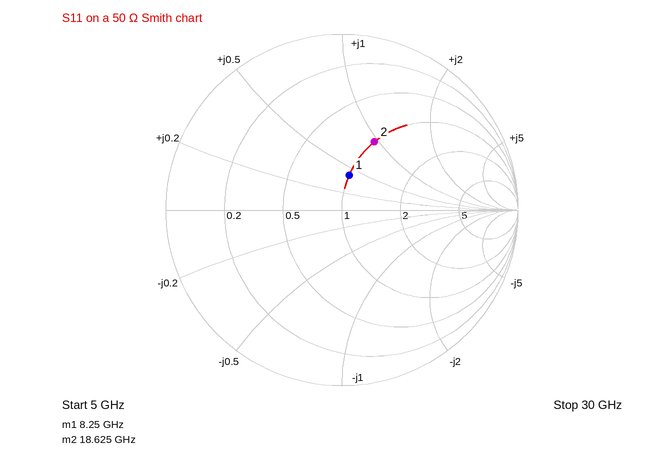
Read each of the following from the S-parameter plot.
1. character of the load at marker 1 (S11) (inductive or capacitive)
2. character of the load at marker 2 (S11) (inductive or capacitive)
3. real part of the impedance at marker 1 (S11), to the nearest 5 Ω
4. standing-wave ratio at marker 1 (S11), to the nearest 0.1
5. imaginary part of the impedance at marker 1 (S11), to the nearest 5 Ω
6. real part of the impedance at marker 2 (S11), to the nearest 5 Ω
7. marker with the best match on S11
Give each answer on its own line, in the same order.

inductive
inductive
50 Ω
1.5
+20 Ω
50 Ω
marker 1
